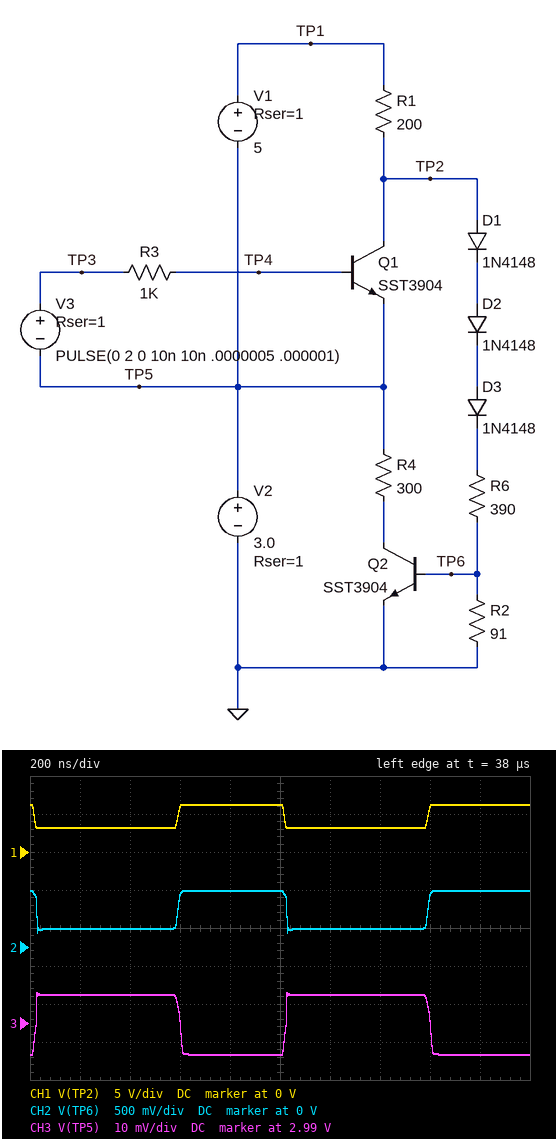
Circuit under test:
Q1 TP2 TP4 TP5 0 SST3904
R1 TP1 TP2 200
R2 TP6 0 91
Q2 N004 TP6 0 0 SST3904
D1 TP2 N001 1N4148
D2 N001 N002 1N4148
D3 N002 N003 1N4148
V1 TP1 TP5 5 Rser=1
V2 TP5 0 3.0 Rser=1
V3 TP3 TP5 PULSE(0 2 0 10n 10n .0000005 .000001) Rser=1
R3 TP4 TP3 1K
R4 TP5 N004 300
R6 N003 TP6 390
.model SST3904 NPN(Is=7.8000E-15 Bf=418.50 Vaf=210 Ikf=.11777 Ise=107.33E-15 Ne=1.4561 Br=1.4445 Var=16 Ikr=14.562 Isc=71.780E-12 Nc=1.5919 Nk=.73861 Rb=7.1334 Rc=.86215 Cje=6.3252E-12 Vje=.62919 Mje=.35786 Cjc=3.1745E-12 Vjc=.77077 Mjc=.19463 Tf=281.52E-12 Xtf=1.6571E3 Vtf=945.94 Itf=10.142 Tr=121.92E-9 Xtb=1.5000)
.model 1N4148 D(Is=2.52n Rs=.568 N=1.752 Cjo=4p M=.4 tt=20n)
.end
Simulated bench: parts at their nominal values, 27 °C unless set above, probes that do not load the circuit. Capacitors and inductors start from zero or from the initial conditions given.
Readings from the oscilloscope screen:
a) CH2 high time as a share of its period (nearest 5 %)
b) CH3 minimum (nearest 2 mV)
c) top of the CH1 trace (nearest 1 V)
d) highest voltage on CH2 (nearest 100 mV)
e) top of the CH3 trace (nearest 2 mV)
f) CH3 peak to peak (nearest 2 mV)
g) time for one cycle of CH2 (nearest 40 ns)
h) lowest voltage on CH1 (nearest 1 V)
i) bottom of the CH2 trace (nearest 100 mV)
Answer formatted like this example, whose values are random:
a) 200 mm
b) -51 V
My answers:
a) 45 %
b) 2.982 V
c) 6 V
d) 700 mV
e) 2.998 V
f) 16 mV
g) 1.00 µs
h) 3 V
i) 200 mV
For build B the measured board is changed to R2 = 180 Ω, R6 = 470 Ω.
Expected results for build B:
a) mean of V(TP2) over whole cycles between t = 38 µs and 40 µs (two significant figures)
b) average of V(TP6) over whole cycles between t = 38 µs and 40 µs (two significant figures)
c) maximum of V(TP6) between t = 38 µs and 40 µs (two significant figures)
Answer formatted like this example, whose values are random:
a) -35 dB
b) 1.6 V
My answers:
a) 4.5 V
b) 560 mV
c) 760 mV
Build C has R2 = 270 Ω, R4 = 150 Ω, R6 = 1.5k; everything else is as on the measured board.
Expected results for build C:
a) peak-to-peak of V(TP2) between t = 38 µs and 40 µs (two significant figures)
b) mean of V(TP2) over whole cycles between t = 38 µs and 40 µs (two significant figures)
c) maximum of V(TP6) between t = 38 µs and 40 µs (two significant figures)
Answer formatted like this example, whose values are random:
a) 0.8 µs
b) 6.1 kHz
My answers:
a) 4.3 V
b) 4.9 V
c) 750 mV
